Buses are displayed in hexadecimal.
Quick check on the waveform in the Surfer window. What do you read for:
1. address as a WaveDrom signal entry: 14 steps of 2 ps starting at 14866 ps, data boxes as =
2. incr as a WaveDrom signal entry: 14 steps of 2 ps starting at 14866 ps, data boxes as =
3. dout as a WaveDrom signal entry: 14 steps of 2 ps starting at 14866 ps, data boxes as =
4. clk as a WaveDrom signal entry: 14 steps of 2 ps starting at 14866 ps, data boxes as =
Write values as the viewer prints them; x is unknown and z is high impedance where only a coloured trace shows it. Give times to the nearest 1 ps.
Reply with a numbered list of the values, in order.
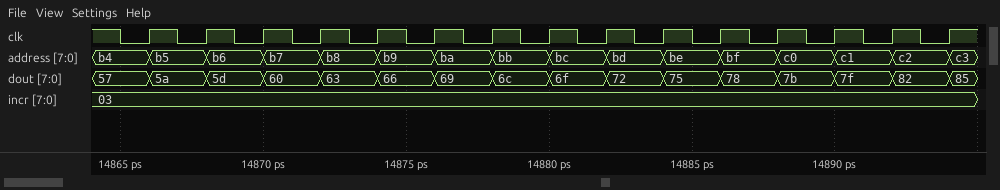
1. {name: 'address', wave: '==============', data: 'b5 b6 b7 b8 b9 ba bb bc bd be bf c0 c1 c2'}
2. {name: 'incr', wave: '=.............', data: '03'}
3. {name: 'dout', wave: '==============', data: '5a 5d 60 63 66 69 6c 6f 72 75 78 7b 7f 82'}
4. {name: 'clk', wave: 'p.............'}
